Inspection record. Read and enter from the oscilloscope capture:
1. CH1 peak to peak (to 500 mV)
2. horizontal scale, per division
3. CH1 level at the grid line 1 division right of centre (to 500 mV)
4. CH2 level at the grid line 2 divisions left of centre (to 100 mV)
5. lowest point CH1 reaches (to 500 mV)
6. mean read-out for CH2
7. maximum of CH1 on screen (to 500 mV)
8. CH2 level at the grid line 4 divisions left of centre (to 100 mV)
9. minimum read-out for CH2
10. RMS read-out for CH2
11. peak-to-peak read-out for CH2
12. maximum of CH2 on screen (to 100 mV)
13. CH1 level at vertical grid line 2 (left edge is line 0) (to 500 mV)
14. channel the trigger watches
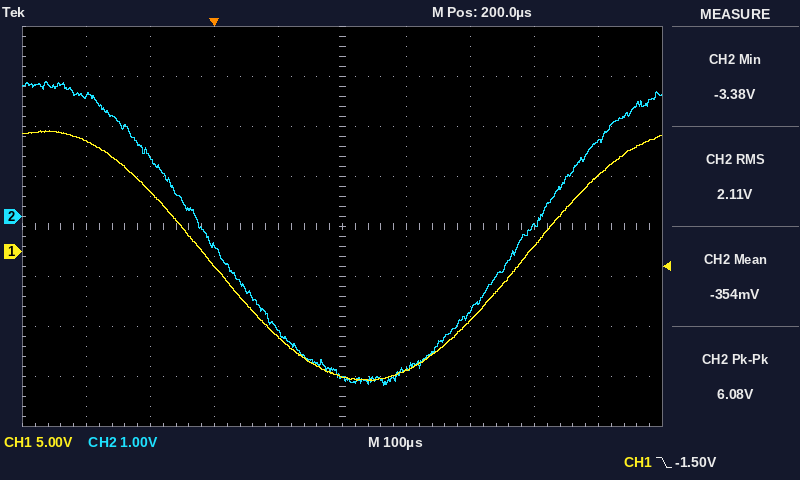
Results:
25.0 V
100 µs
-12.0 V
-600 mV
-13.0 V
-354 mV
12.0 V
2.4 V
-3.38 V
2.11 V
6.08 V
2.7 V
6.0 V
CH1
